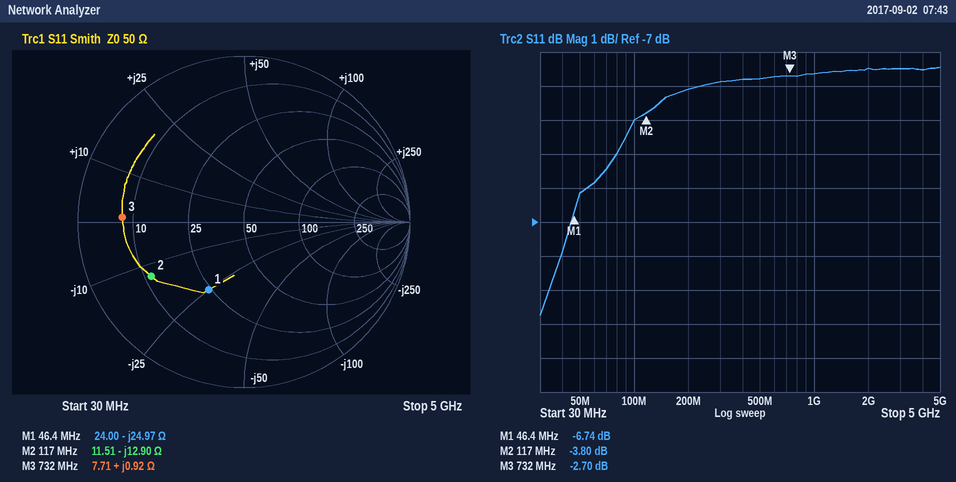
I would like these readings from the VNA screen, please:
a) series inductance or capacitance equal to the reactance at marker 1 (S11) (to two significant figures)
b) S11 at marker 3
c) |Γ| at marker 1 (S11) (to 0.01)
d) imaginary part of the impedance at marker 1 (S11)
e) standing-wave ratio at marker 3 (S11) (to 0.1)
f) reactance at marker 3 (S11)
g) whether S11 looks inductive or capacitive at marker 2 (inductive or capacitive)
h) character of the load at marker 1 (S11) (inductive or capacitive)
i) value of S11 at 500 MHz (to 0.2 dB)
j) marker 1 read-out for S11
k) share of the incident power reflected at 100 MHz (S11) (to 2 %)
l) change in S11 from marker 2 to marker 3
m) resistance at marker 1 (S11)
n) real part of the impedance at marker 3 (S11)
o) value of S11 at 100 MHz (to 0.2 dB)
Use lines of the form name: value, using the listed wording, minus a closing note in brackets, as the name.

series inductance or capacitance equal to the reactance at marker 1 (S11): 140 pF
S11 at marker 3: -2.70 dB
|Γ| at marker 1 (S11): 0.46
imaginary part of the impedance at marker 1: -24.97 Ω
standing-wave ratio at marker 3 (S11): 6.5
reactance at marker 3: +0.92 Ω
whether S11 looks inductive or capacitive at marker 2: capacitive
character of the load at marker 1 (S11): capacitive
value of S11 at 500 MHz: -2.8 dB
marker 1 read-out for S11: -6.74 dB
share of the incident power reflected at 100 MHz (S11): 40 %
change in S11 from marker 2 to marker 3: 1.10 dB
resistance at marker 1: 24.00 Ω
real part of the impedance at marker 3: 7.71 Ω
value of S11 at 100 MHz: -4.0 dB
